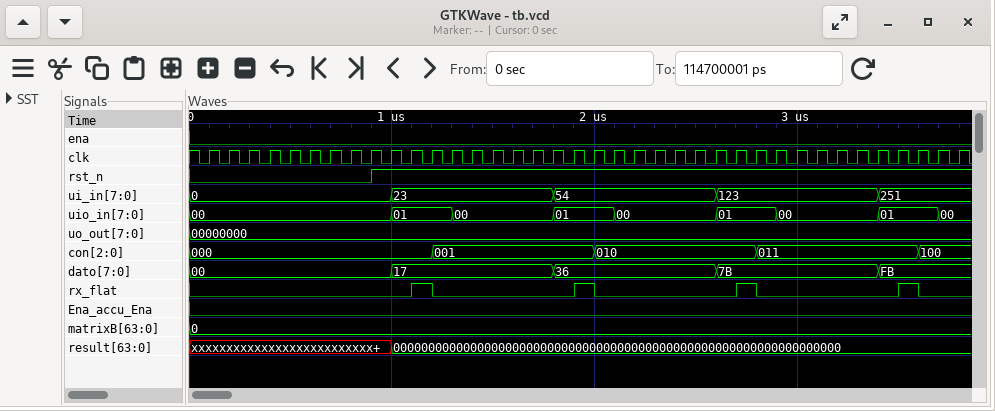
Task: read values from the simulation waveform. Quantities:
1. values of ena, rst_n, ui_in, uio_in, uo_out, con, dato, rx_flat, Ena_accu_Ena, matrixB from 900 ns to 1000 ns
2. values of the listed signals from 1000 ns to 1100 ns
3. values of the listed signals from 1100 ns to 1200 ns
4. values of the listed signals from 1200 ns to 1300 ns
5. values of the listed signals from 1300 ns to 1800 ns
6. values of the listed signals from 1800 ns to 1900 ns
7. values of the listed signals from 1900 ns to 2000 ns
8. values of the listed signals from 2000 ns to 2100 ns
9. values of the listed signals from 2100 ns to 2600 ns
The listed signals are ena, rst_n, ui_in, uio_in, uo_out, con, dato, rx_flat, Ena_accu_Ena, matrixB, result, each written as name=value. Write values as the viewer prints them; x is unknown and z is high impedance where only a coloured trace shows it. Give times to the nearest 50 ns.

ena=0, rst_n=1, ui_in=0, uio_in=00, uo_out=00000000, con=000, dato=00, rx_flat=0, Ena_accu_Ena=0, matrixB=0
ena=0, rst_n=1, ui_in=23, uio_in=01, uo_out=00000000, con=000, dato=17, rx_flat=0, Ena_accu_Ena=0, matrixB=0, result=0000000000000000000000000000000000000000000000000000000000000000
ena=0, rst_n=1, ui_in=23, uio_in=01, uo_out=00000000, con=000, dato=17, rx_flat=1, Ena_accu_Ena=0, matrixB=0, result=0000000000000000000000000000000000000000000000000000000000000000
ena=0, rst_n=1, ui_in=23, uio_in=01, uo_out=00000000, con=001, dato=17, rx_flat=0, Ena_accu_Ena=0, matrixB=0, result=0000000000000000000000000000000000000000000000000000000000000000
ena=0, rst_n=1, ui_in=23, uio_in=00, uo_out=00000000, con=001, dato=17, rx_flat=0, Ena_accu_Ena=0, matrixB=0, result=0000000000000000000000000000000000000000000000000000000000000000
ena=0, rst_n=1, ui_in=54, uio_in=01, uo_out=00000000, con=001, dato=36, rx_flat=0, Ena_accu_Ena=0, matrixB=0, result=0000000000000000000000000000000000000000000000000000000000000000
ena=0, rst_n=1, ui_in=54, uio_in=01, uo_out=00000000, con=001, dato=36, rx_flat=1, Ena_accu_Ena=0, matrixB=0, result=0000000000000000000000000000000000000000000000000000000000000000
ena=0, rst_n=1, ui_in=54, uio_in=01, uo_out=00000000, con=010, dato=36, rx_flat=0, Ena_accu_Ena=0, matrixB=0, result=0000000000000000000000000000000000000000000000000000000000000000
ena=0, rst_n=1, ui_in=54, uio_in=00, uo_out=00000000, con=010, dato=36, rx_flat=0, Ena_accu_Ena=0, matrixB=0, result=0000000000000000000000000000000000000000000000000000000000000000
